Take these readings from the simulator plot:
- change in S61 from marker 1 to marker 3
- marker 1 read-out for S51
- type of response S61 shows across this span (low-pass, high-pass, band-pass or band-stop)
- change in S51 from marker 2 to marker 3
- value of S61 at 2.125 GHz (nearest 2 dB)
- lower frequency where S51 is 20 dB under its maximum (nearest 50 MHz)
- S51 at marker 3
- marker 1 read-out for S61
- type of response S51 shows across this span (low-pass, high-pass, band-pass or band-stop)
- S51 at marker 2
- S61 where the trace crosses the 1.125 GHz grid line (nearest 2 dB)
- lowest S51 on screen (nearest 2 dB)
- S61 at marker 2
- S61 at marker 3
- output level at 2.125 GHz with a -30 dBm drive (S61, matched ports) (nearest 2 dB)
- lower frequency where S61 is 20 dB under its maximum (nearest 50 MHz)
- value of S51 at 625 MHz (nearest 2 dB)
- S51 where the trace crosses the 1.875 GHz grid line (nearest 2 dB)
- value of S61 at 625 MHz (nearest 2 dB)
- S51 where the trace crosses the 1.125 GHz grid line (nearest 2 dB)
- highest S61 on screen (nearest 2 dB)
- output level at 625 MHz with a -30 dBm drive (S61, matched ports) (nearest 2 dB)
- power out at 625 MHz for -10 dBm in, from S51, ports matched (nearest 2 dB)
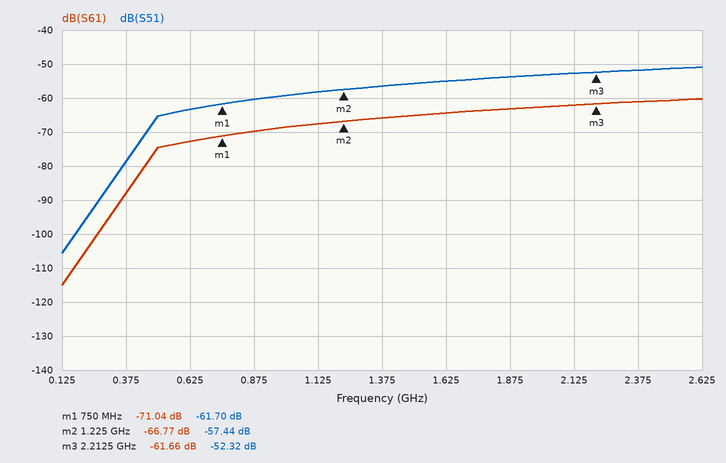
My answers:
9.38 dB
-61.70 dB
high-pass
5.12 dB
-62 dB
450 MHz
-52.32 dB
-71.04 dB
high-pass
-57.44 dB
-68 dB
-106 dB
-66.77 dB
-61.66 dB
-92 dBm
450 MHz
-64 dB
-54 dB
-72 dB
-58 dB
-60 dB
-102 dBm
-74 dBm
